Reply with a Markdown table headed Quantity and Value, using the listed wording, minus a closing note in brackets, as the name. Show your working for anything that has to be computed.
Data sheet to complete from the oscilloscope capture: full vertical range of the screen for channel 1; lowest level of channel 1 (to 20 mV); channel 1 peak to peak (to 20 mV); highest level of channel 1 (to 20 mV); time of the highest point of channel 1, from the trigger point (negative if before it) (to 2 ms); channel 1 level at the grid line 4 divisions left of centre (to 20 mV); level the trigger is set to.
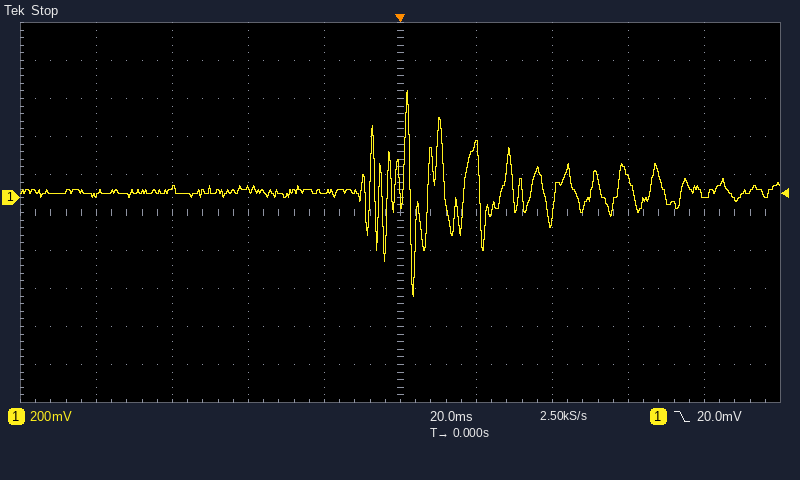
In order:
| Quantity | Value |
|---|---|
| full vertical range of the screen for channel 1 | 2 V |
| lowest level of channel 1 | -520 mV |
| channel 1 peak to peak | 560 mV − (-520 mV) = 1.08 V |
| highest level of channel 1 | 560 mV |
| time of the highest point of channel 1, from the trigger point (negative if before it) | +2 ms |
| channel 1 level at the grid line 4 divisions left of centre | 20 mV |
| level the trigger is set to | 20.0 mV |
